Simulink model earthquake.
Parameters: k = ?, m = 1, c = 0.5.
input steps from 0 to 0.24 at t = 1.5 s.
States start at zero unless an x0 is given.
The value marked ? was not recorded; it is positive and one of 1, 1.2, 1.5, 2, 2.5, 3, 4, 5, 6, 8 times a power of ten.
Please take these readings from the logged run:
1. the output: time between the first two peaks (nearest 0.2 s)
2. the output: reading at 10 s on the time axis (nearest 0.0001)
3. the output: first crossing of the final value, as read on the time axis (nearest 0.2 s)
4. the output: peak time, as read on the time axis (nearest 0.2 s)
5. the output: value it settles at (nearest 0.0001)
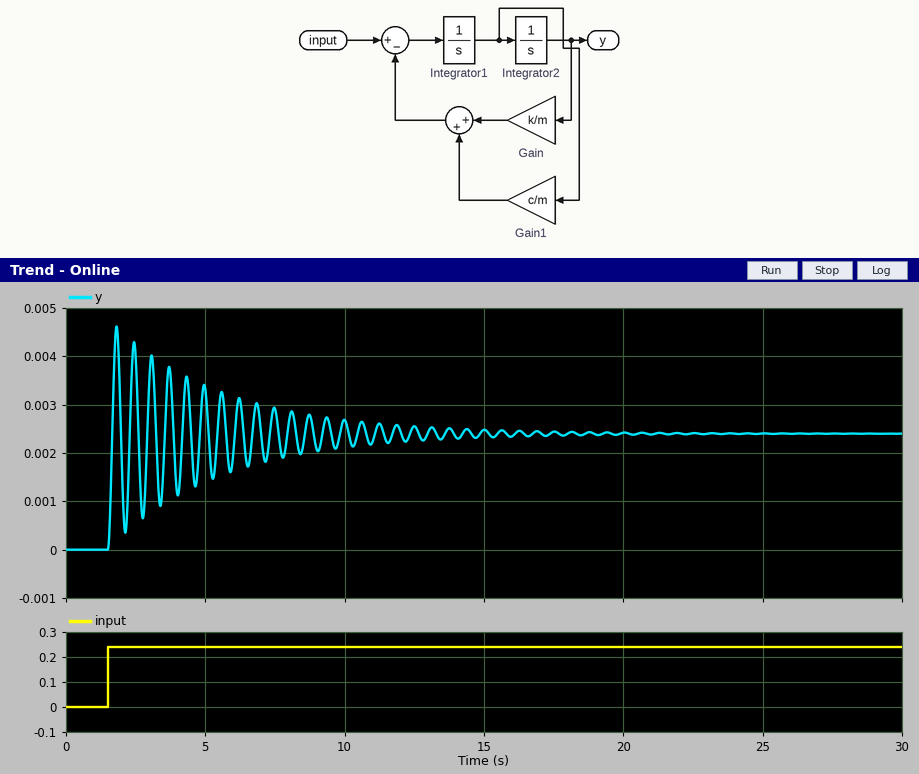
0.6 s
0.0027
1.6 s
1.8 s
0.0024
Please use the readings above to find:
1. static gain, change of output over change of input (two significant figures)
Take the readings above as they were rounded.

0.010
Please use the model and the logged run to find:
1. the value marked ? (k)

100
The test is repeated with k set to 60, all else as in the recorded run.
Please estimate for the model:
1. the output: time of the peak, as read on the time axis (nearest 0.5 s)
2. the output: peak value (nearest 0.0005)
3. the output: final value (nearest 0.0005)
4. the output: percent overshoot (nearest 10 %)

2.0 s
0.0075
0.0040
90 %
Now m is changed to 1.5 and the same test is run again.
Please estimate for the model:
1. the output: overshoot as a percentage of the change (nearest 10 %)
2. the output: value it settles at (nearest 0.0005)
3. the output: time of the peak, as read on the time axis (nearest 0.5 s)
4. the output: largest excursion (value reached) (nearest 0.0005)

90 %
0.0035
2.0 s
0.0070
